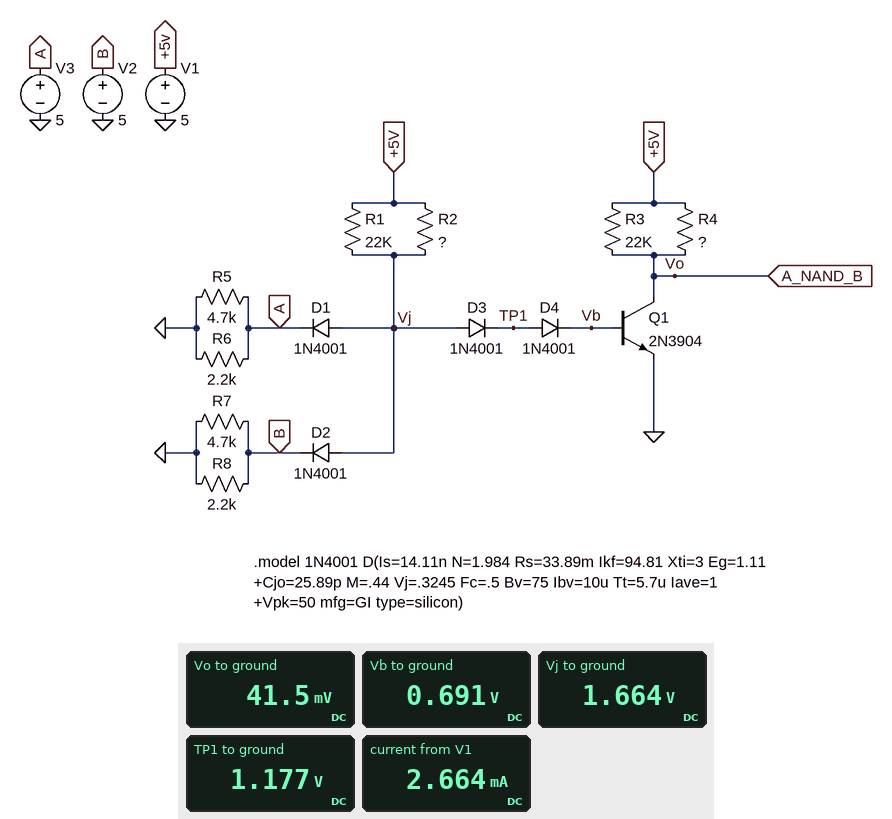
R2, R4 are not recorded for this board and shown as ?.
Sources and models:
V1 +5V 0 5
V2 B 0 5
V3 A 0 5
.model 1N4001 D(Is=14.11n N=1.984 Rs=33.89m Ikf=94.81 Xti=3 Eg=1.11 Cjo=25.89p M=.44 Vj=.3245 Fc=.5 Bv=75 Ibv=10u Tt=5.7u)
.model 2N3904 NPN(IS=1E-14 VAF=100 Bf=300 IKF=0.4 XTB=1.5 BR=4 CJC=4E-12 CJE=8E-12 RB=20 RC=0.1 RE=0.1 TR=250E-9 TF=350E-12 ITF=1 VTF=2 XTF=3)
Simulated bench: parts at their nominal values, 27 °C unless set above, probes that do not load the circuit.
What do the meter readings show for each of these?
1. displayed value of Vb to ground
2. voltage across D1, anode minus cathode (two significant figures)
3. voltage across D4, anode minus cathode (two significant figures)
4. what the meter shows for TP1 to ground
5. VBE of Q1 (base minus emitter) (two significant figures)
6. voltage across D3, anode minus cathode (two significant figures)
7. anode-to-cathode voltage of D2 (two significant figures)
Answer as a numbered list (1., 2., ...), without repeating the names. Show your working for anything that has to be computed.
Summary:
1. 0.691 V
2. 1.664 V - 5 V = -3.3 V
3. 1.177 V - 691 mV = 490 mV
4. 1.177 V
5. 691 mV = 690 mV
6. 1.664 V - 1.177 V = 490 mV
7. 1.664 V - 5 V = -3.3 V
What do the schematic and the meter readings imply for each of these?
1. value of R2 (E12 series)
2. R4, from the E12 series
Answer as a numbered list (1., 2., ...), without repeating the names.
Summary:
1. 100 kΩ
2. 2.2 kΩ
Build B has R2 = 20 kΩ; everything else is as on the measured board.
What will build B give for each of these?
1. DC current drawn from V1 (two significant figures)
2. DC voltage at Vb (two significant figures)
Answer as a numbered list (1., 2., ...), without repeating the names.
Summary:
1. 2.8 mA
2. 700 mV
